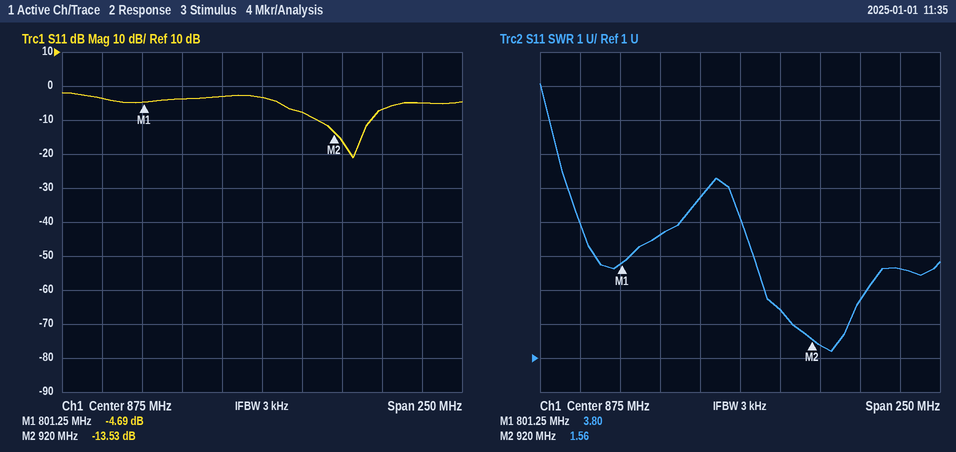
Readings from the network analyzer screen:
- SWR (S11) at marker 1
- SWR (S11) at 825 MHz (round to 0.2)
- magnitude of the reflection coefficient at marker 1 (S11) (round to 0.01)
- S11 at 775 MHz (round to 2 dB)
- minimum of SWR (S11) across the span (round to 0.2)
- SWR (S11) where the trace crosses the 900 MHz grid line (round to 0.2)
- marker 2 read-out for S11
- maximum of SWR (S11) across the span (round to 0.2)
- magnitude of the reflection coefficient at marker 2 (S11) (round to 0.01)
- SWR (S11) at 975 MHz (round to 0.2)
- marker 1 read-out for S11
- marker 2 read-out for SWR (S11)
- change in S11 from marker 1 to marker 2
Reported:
3.80
4.6
0.58
-4 dB
1.2
2.4
-13.53 dB
9.0
0.21
3.6
-4.69 dB
1.56
-8.84 dB
